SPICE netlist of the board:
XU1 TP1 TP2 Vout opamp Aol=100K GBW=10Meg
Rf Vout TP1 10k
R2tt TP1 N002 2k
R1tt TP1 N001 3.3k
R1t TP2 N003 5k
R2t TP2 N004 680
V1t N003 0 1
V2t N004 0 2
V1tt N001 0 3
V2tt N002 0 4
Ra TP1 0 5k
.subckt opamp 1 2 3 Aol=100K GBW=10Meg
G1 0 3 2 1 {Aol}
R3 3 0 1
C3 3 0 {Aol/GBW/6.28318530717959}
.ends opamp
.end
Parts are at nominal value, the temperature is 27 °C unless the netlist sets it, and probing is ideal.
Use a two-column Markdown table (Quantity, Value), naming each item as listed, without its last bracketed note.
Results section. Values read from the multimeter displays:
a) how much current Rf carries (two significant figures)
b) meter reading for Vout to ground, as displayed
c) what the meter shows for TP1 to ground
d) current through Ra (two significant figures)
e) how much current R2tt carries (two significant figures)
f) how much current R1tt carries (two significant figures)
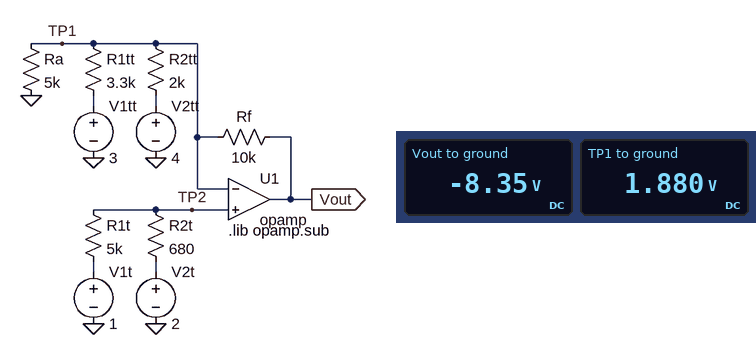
| Quantity | Value |
|---|---|
| how much current Rf carries | 1.0 mA |
| meter reading for Vout to ground, as displayed | -8.35 V |
| what the meter shows for TP1 to ground | 1.880 V |
| current through Ra | 380 µA |
| how much current R2tt carries | 1.1 mA |
| how much current R1tt carries | 340 µA |
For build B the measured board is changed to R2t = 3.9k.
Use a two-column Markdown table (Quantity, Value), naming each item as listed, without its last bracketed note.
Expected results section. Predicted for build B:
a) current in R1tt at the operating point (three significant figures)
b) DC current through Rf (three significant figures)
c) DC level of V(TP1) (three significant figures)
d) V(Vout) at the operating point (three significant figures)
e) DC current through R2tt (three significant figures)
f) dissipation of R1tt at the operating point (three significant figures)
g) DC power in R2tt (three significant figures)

| Quantity | Value |
|---|---|
| current in R1tt at the operating point | 436 µA |
| DC current through Rf | 1.34 mA |
| DC level of V(TP1) | 1.56 V |
| V(Vout) at the operating point | -11.9 V |
| DC current through R2tt | 1.22 mA |
| dissipation of R1tt at the operating point | 627 µW |
| DC power in R2tt | 2.97 mW |
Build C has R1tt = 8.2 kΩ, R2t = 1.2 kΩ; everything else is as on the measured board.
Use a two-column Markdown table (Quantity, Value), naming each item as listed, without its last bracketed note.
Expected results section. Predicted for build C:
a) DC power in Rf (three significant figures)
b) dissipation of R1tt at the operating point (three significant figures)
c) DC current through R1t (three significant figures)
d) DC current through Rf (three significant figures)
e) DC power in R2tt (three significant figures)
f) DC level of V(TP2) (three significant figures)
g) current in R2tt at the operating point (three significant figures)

| Quantity | Value |
|---|---|
| DC power in Rf | 7.76 mW |
| dissipation of R1tt at the operating point | 174 µW |
| DC current through R1t | 161 µA |
| DC current through Rf | 881 µA |
| DC power in R2tt | 2.41 mW |
| DC level of V(TP2) | 1.81 V |
| current in R2tt at the operating point | 1.10 mA |
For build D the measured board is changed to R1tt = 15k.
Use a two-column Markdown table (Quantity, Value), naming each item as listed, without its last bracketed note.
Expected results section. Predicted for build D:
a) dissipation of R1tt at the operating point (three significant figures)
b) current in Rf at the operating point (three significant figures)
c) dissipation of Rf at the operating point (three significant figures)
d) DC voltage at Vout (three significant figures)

| Quantity | Value |
|---|---|
| dissipation of R1tt at the operating point | 83.6 µW |
| current in Rf at the operating point | 758 µA |
| dissipation of Rf at the operating point | 5.75 mW |
| DC voltage at Vout | -5.70 V |
